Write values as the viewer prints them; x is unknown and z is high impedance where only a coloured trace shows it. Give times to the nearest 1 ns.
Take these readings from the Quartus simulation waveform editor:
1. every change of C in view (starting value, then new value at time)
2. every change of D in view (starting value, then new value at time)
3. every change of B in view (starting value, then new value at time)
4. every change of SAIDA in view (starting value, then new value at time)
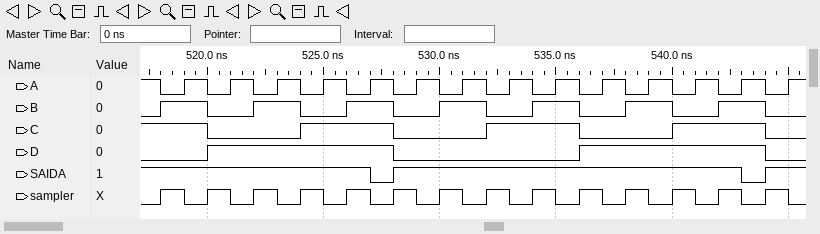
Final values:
1, 0 at 520 ns, 1 at 524 ns, 0 at 528 ns, 1 at 532 ns, 0 at 536 ns, 1 at 540 ns, 0 at 544 ns
0, 1 at 520 ns, 0 at 528 ns, 1 at 536 ns, 0 at 544 ns
0, 1 at 518 ns, 0 at 520 ns, 1 at 522 ns, 0 at 524 ns, 1 at 526 ns, 0 at 528 ns, 1 at 530 ns, 0 at 532 ns, 1 at 534 ns, 0 at 536 ns, 1 at 538 ns, 0 at 540 ns, 1 at 542 ns, 0 at 544 ns
1, 0 at 527 ns, 1 at 528 ns, 0 at 543 ns, 1 at 544 ns
